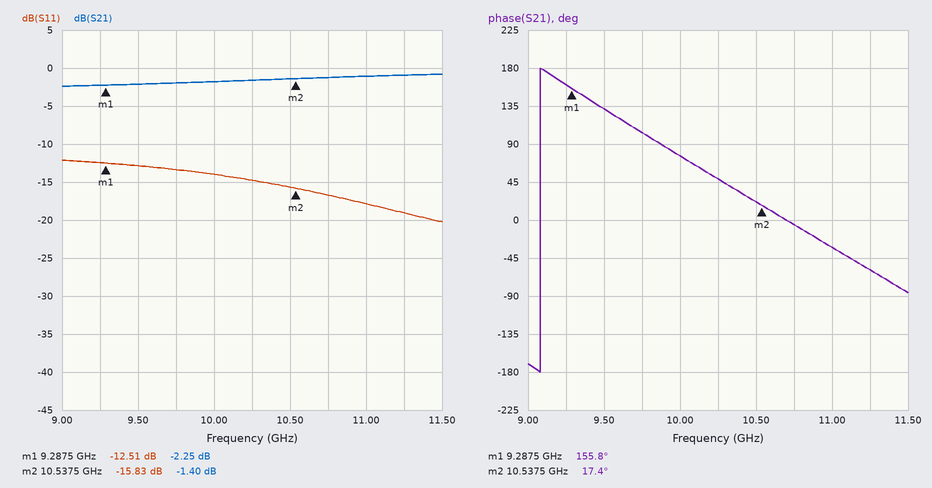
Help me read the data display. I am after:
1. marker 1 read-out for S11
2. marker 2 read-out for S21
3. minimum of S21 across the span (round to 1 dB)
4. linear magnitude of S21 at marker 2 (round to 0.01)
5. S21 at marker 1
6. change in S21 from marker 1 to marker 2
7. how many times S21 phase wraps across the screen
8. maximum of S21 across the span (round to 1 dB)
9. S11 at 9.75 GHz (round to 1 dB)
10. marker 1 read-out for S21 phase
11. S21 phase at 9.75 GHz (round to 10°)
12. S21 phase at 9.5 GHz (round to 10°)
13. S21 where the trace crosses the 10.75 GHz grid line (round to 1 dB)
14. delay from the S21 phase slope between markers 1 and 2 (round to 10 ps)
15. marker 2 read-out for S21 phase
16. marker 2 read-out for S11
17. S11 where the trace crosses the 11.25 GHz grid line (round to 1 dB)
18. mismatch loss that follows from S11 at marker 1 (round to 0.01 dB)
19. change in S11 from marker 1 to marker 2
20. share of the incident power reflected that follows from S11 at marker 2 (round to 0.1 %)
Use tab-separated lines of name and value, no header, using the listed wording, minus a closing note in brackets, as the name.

marker 1 read-out for S11	-12.51 dB
marker 2 read-out for S21	-1.40 dB
minimum of S21 across the span	-2 dB
linear magnitude of S21 at marker 2	0.85
S21 at marker 1	-2.25 dB
change in S21 from marker 1 to marker 2	0.85 dB
how many times S21 phase wraps across the screen	1
maximum of S21 across the span	-1 dB
S11 at 9.75 GHz	-13 dB
marker 1 read-out for S21 phase	155.8°
S21 phase at 9.75 GHz	100°
S21 phase at 9.5 GHz	130°
S21 where the trace crosses the 10.75 GHz grid line	-1 dB
delay from the S21 phase slope between markers 1 and 2	310 ps
marker 2 read-out for S21 phase	17.4°
marker 2 read-out for S11	-15.83 dB
S11 where the trace crosses the 11.25 GHz grid line	-19 dB
mismatch loss that follows from S11 at marker 1	0.25 dB
change in S11 from marker 1 to marker 2	-3.32 dB
share of the incident power reflected that follows from S11 at marker 2	2.6 %
